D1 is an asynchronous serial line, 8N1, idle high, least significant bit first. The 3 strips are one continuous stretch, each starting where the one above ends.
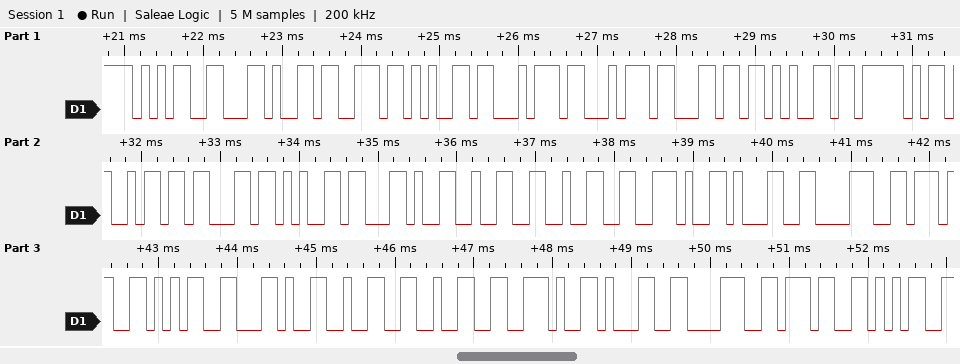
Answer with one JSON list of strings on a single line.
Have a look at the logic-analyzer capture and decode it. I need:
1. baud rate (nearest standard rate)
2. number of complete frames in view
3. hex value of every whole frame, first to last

["9600 baud", "28", "35 2C 73 65 74 74 6C 65 5F 69 63 65 2C 32 32 2E 31 38 37 35 2C 32 32 2E 31 38 37 35"]
